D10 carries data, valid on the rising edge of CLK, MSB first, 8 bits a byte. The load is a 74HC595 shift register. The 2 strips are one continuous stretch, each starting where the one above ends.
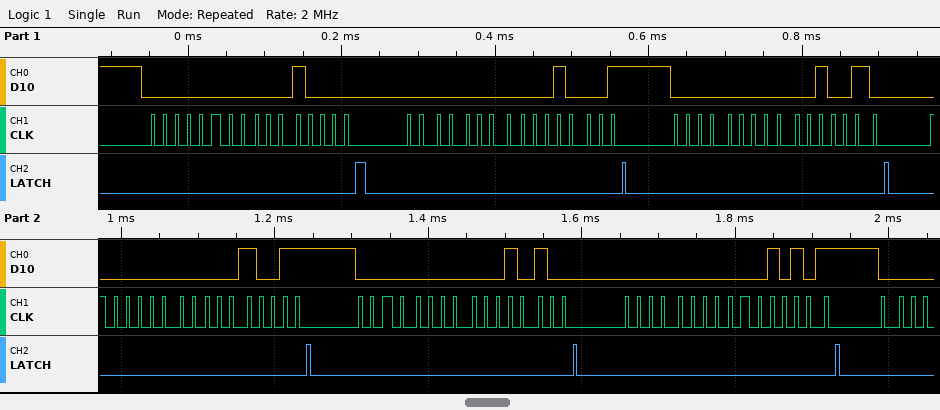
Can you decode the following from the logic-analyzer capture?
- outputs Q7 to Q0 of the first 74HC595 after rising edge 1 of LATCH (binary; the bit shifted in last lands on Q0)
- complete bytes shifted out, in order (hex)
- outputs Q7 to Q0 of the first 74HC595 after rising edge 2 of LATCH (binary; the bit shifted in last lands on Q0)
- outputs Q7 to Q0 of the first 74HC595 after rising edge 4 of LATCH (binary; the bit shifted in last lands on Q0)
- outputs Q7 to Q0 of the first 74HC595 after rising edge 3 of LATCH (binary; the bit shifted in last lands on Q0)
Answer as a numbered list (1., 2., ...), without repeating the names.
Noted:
1. 00010000
2. 0x00 0x10 0x00 0x11 0x00 0x12 0x00 0x13 0x00 0x14 0x00 0x15
3. 00010001
4. 00010011
5. 00010010
